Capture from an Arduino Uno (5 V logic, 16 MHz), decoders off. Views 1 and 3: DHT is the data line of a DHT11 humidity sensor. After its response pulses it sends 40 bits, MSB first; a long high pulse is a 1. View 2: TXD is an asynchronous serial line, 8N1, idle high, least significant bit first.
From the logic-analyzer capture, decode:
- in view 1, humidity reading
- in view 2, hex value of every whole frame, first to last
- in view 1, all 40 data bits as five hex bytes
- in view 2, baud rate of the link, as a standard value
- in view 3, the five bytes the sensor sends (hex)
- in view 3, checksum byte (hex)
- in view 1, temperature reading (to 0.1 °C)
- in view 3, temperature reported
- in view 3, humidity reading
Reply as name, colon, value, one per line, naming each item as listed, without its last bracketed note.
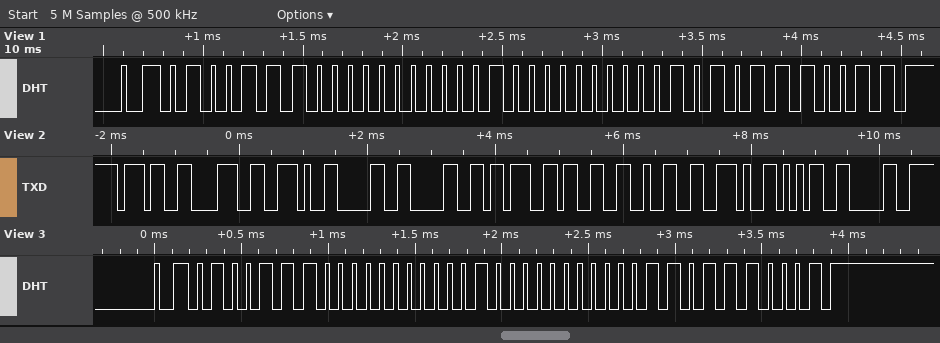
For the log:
in view 1, humidity reading: 78 %
in view 2, hex value of every whole frame, first to last: 0x37 0x38 0x2E 0x30 0x30 0x3B 0x33 0x32 0x2E 0x35 0x30
in view 1, all 40 data bits as five hex bytes: 4E 00 20 05 73
in view 2, baud rate of the link, as a standard value: 9600 baud
in view 3, the five bytes the sensor sends: 4E 00 20 03 71
in view 3, checksum byte: 0x71
in view 1, temperature reading: 32.5 °C
in view 3, temperature reported: 32.3 °C
in view 3, humidity reading: 78 %
